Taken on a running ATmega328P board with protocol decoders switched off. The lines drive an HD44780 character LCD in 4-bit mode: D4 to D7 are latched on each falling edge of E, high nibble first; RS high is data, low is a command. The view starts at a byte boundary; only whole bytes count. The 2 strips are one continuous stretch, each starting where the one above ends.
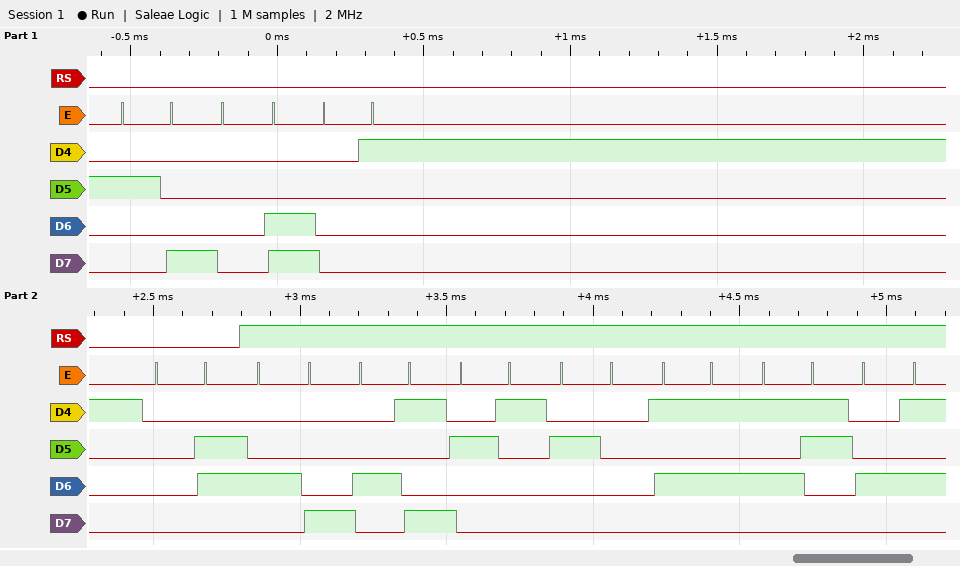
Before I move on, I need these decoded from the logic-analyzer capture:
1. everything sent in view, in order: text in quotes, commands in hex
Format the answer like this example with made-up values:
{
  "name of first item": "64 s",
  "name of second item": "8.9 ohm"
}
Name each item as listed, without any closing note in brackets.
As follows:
{
  "everything sent in view, in order: text in quotes, commands in hex": "0x28 0x0C 0x01 0x06 \"HI! USE\""
}
